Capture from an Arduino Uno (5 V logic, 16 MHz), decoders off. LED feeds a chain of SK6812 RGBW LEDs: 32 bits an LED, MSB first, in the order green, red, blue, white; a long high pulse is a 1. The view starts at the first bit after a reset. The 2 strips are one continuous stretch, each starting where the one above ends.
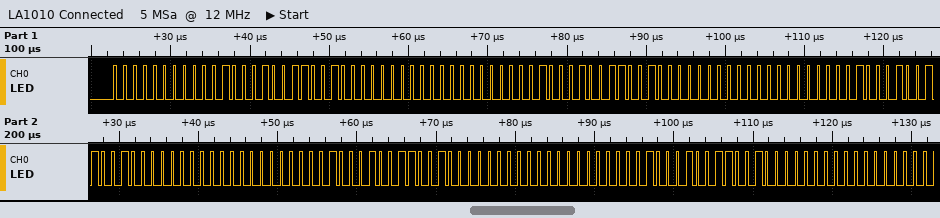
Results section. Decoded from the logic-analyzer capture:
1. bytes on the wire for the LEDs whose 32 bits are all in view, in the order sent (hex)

00 11 32 00 00 11 32 00 00 11 32 00 00 11 32 00 00 11 32 00
